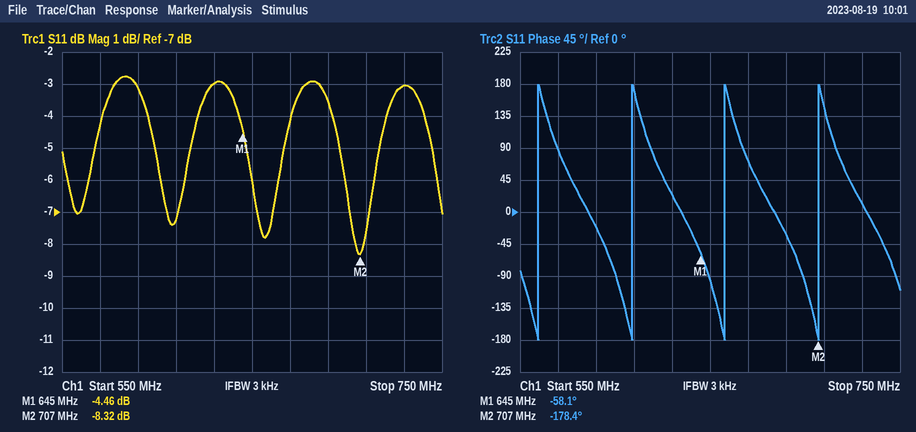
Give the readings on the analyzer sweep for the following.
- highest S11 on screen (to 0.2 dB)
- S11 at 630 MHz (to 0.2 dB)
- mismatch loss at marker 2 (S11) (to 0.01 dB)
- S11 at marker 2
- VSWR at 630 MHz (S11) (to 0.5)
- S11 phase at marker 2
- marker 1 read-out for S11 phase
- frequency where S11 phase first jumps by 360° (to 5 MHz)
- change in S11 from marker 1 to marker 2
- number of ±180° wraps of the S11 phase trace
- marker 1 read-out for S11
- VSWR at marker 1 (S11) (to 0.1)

-2.8 dB
-3.0 dB
0.69 dB
-8.32 dB
6.0
-178.4°
-58.1°
560 MHz
-3.86 dB
4
-4.46 dB
4.0
